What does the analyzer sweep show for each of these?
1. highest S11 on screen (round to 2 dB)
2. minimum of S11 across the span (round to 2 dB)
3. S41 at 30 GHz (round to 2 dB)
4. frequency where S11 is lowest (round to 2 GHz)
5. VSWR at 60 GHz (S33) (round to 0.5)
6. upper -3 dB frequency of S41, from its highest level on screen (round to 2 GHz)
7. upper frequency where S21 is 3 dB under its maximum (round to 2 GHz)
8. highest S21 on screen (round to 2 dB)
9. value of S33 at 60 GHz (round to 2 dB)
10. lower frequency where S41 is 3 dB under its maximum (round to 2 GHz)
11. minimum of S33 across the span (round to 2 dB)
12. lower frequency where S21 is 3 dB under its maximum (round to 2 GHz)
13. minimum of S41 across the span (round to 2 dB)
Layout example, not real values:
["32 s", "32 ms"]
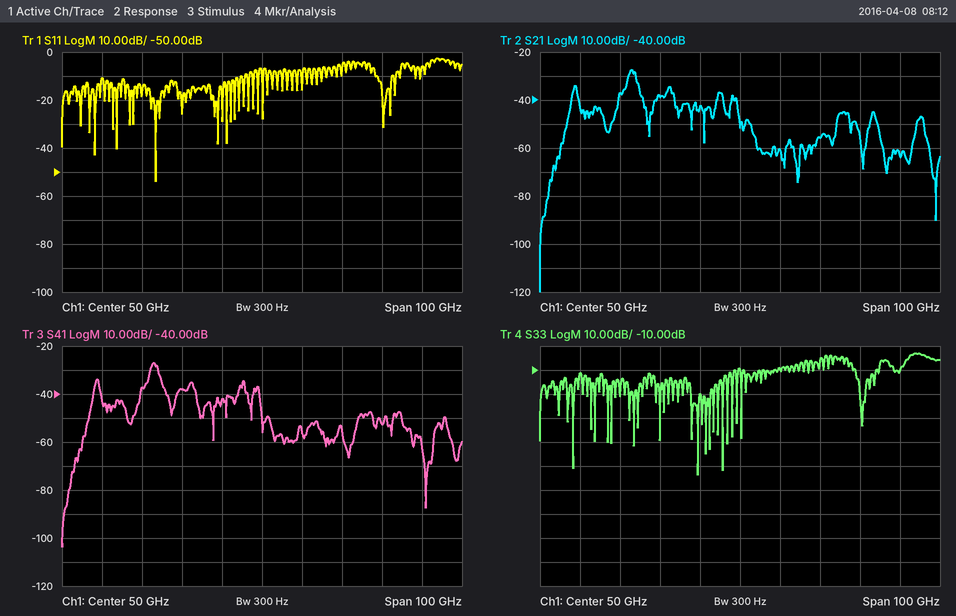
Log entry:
["-2 dB", "-54 dB", "-38 dB", "24 GHz", "2.0", "24 GHz", "24 GHz", "-28 dB", "-10 dB", "22 GHz", "-54 dB", "22 GHz", "-104 dB"]
